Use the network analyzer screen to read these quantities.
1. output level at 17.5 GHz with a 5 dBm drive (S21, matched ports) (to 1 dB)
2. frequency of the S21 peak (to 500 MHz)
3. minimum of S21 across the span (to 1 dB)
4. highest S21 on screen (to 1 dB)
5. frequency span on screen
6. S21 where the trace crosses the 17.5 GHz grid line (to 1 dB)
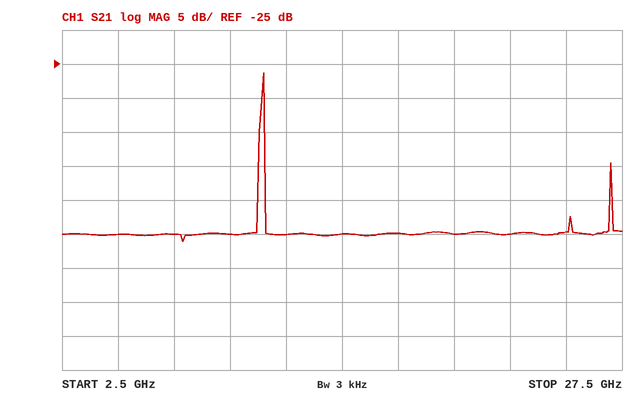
-45 dBm
11.5 GHz
-51 dB
-26 dB
25 GHz
-50 dB
